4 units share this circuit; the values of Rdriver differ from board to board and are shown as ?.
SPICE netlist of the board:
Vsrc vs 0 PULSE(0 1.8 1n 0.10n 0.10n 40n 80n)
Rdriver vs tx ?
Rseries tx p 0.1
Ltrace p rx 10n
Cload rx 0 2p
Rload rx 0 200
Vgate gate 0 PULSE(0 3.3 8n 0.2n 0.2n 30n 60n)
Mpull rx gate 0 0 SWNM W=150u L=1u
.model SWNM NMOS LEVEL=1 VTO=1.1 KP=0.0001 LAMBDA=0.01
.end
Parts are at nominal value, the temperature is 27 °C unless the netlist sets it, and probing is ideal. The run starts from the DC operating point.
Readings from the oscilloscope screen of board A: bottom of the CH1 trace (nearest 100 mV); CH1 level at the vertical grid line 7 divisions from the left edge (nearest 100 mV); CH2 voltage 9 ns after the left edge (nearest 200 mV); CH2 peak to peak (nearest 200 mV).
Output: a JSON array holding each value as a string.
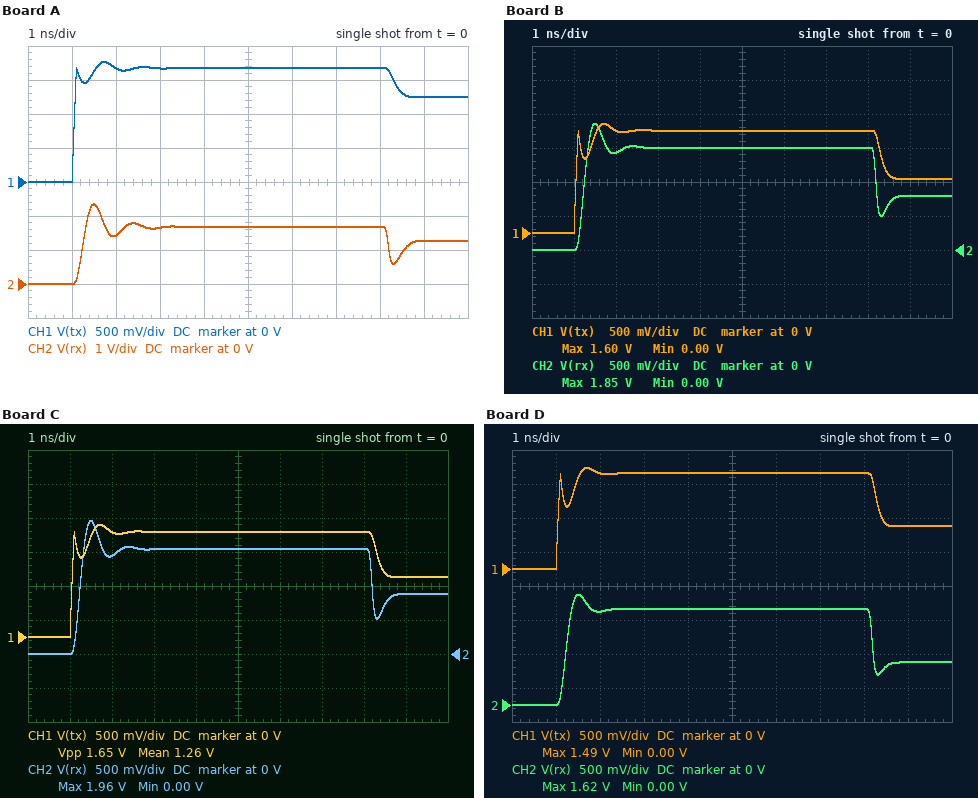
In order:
["0 V", "1.7 V", "1.2 V", "2.4 V"]
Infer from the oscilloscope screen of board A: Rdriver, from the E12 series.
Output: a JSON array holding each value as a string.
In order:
["15 Ω"]
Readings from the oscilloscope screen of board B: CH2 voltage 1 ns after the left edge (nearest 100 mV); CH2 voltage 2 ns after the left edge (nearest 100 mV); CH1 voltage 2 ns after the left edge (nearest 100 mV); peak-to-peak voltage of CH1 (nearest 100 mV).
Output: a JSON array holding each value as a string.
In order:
["0 V", "1.4 V", "1.5 V", "1.6 V"]
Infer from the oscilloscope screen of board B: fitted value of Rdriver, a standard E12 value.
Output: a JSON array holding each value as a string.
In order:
["39 Ω"]
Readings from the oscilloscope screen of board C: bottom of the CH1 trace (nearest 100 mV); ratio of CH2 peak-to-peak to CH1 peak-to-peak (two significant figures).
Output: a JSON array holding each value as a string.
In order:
["0 V", "1.2"]
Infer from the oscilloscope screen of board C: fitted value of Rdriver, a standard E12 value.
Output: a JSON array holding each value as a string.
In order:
["33 Ω"]
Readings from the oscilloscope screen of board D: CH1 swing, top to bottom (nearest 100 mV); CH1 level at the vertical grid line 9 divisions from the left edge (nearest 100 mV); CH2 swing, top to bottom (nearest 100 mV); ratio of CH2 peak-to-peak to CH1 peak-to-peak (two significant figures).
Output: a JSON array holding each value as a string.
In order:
["1.5 V", "600 mV", "1.6 V", "1.1"]
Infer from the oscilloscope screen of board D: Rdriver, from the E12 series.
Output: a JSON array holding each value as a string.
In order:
["56 Ω"]
